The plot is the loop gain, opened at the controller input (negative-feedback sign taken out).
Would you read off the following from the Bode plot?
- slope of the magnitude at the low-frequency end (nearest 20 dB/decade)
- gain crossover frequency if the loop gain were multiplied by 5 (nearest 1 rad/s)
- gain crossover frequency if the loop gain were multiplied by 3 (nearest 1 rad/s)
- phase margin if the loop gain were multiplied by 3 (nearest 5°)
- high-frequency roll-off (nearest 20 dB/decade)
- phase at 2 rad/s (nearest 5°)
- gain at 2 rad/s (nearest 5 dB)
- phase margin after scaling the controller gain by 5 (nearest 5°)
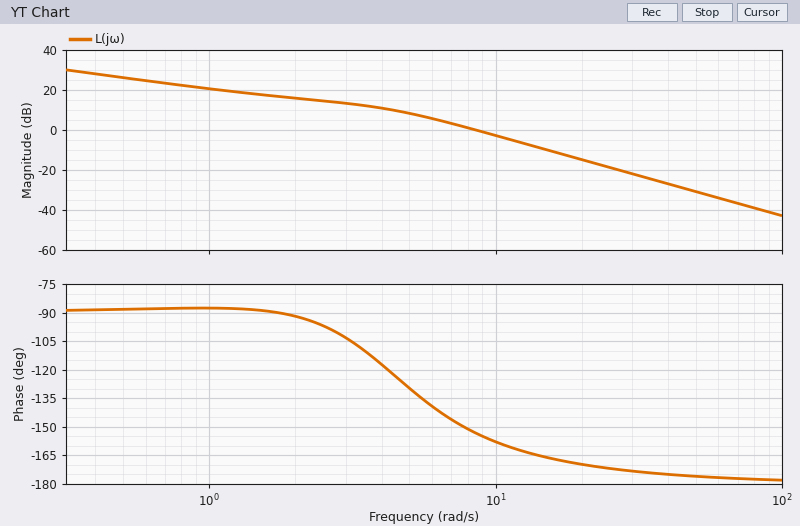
-20 dB/decade
19 rad/s
15 rad/s
15°
-40 dB/decade
-90°
15 dB
10°
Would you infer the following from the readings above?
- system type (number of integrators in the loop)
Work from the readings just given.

1
